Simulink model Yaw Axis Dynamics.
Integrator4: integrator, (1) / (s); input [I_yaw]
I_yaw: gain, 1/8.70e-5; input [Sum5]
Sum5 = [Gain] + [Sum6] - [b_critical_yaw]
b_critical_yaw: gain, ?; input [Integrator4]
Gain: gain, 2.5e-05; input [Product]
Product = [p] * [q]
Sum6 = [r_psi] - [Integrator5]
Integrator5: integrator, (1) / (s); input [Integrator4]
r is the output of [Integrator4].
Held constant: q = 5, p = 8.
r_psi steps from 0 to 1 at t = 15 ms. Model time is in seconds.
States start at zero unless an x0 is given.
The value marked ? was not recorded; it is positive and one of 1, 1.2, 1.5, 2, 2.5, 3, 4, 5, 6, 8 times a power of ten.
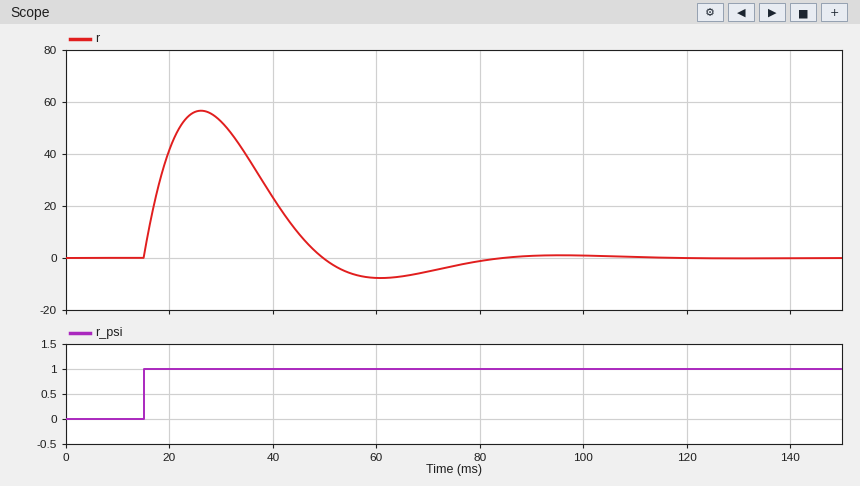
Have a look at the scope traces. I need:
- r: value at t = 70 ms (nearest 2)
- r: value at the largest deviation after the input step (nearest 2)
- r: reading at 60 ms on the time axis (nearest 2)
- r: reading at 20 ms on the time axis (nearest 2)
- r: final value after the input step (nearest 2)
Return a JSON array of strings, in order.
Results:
["-6", "56", "-8", "42", "0"]
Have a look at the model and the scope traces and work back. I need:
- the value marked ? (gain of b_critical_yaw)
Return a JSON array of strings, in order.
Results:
["0.01"]
